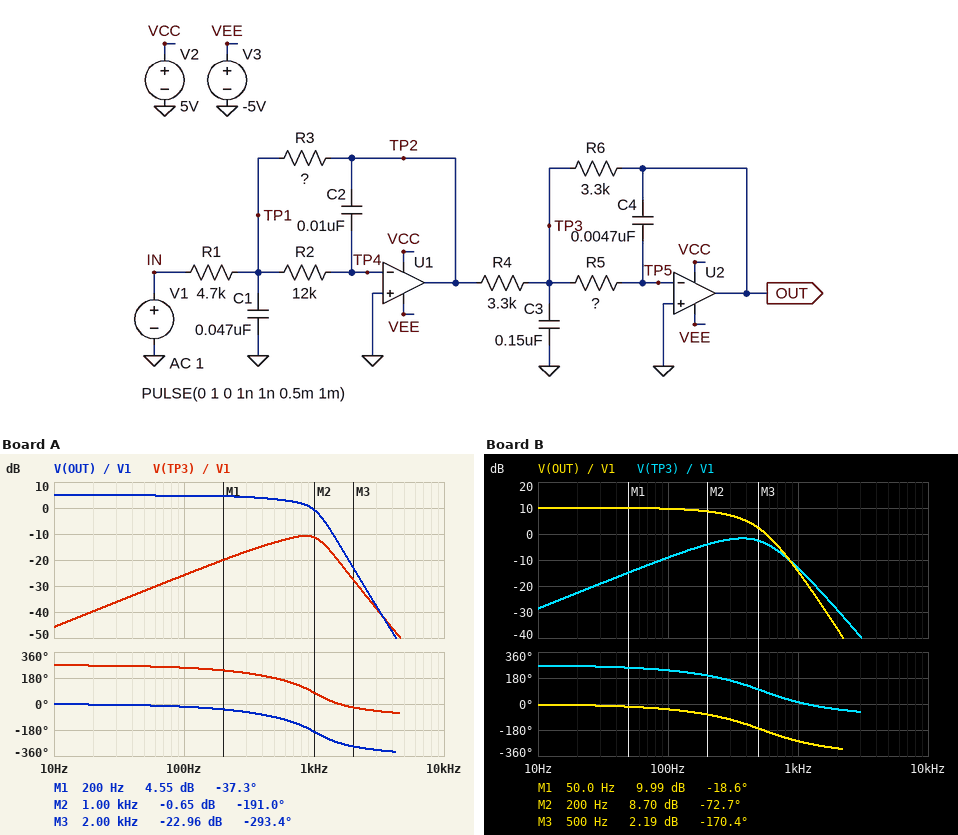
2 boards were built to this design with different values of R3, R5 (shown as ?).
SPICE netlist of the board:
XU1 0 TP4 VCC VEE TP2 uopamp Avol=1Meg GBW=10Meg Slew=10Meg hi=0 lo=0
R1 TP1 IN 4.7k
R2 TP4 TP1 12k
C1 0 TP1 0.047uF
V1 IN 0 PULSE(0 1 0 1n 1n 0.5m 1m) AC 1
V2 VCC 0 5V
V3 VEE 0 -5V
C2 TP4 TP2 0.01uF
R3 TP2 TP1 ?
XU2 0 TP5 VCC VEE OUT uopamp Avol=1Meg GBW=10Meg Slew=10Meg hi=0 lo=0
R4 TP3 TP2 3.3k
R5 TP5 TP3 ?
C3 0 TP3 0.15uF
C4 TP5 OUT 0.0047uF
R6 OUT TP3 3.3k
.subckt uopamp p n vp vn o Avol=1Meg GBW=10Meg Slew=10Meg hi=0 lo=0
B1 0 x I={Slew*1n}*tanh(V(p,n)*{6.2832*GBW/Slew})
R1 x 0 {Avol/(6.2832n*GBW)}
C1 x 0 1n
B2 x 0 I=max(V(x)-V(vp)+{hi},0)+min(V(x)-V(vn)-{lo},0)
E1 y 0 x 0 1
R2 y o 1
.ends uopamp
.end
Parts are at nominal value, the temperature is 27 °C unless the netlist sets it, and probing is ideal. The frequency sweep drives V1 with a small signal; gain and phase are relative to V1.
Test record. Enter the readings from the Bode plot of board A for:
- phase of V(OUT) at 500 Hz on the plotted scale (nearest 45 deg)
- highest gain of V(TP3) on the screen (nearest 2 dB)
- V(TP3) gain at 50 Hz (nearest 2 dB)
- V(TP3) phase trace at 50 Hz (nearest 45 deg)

-90 deg
-10 dB
-32 dB
270 deg
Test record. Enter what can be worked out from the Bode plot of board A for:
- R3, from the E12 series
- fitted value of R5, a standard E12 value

8.2 kΩ
10 kΩ
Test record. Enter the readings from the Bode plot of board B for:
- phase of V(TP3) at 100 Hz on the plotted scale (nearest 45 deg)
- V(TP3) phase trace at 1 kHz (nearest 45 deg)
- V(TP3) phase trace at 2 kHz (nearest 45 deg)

225 deg
0 deg
-45 deg
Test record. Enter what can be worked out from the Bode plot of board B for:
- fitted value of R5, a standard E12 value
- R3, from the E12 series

39 kΩ
15 kΩ
